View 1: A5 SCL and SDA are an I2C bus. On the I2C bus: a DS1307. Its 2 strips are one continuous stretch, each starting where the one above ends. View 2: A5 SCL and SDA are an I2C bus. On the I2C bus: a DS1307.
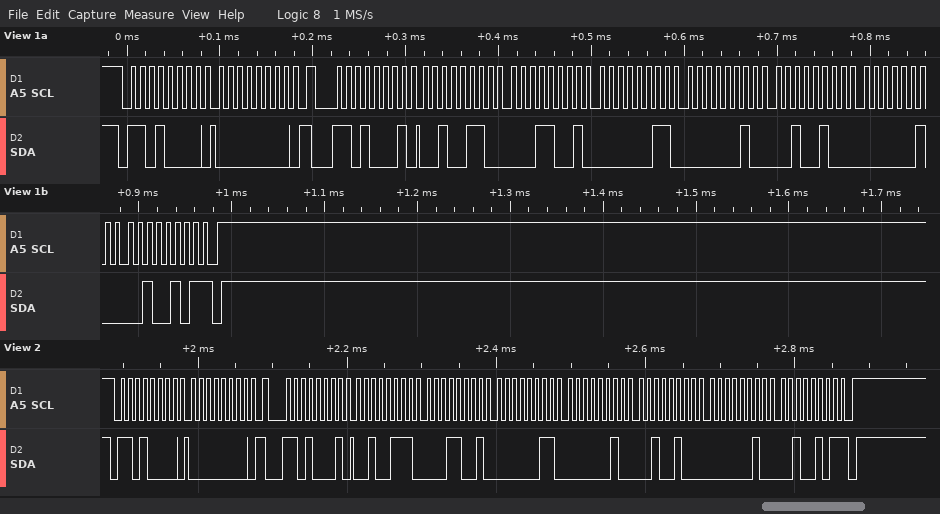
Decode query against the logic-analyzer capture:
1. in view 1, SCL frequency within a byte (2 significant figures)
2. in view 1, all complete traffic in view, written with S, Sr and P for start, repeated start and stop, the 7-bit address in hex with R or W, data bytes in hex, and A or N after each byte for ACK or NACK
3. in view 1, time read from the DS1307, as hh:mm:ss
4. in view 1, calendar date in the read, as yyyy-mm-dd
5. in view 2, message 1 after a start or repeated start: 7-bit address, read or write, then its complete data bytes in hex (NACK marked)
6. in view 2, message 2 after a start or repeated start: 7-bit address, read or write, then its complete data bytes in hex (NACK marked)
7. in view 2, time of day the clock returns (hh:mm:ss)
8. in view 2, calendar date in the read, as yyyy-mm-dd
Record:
100 kHz
S 68W A 00 A Sr 68R A 26 A 19 A 03 A 02 A 24 A 02 A 25 N P
03:19:26
2025-02-24
0x68 write: 00
0x68 read: 27 19 03 02 24 02 25 NACK
03:19:27
2025-02-24
